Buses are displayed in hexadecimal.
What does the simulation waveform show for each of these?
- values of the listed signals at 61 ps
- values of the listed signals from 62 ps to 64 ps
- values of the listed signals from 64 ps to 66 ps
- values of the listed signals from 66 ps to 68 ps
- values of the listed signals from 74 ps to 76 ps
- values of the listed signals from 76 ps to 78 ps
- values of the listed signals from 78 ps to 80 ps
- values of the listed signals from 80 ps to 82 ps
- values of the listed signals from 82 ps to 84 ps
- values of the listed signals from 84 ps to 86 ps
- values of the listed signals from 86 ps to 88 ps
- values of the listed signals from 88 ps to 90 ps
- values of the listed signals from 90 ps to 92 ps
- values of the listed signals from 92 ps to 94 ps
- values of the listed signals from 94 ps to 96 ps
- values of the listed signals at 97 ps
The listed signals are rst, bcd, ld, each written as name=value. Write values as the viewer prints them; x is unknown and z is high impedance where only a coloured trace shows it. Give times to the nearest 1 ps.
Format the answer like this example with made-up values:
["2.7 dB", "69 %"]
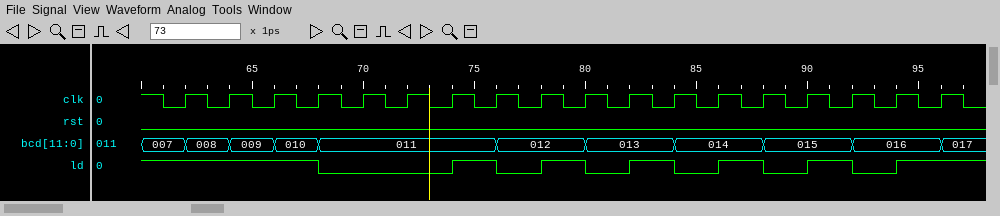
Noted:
["rst=0, bcd=007, ld=1", "rst=0, bcd=008, ld=1", "rst=0, bcd=009, ld=1", "rst=0, bcd=010, ld=1", "rst=0, bcd=011, ld=1", "rst=0, bcd=012, ld=0", "rst=0, bcd=012, ld=1", "rst=0, bcd=013, ld=0", "rst=0, bcd=013, ld=1", "rst=0, bcd=014, ld=0", "rst=0, bcd=014, ld=1", "rst=0, bcd=015, ld=0", "rst=0, bcd=015, ld=1", "rst=0, bcd=016, ld=0", "rst=0, bcd=016, ld=1", "rst=0, bcd=017, ld=1"]
